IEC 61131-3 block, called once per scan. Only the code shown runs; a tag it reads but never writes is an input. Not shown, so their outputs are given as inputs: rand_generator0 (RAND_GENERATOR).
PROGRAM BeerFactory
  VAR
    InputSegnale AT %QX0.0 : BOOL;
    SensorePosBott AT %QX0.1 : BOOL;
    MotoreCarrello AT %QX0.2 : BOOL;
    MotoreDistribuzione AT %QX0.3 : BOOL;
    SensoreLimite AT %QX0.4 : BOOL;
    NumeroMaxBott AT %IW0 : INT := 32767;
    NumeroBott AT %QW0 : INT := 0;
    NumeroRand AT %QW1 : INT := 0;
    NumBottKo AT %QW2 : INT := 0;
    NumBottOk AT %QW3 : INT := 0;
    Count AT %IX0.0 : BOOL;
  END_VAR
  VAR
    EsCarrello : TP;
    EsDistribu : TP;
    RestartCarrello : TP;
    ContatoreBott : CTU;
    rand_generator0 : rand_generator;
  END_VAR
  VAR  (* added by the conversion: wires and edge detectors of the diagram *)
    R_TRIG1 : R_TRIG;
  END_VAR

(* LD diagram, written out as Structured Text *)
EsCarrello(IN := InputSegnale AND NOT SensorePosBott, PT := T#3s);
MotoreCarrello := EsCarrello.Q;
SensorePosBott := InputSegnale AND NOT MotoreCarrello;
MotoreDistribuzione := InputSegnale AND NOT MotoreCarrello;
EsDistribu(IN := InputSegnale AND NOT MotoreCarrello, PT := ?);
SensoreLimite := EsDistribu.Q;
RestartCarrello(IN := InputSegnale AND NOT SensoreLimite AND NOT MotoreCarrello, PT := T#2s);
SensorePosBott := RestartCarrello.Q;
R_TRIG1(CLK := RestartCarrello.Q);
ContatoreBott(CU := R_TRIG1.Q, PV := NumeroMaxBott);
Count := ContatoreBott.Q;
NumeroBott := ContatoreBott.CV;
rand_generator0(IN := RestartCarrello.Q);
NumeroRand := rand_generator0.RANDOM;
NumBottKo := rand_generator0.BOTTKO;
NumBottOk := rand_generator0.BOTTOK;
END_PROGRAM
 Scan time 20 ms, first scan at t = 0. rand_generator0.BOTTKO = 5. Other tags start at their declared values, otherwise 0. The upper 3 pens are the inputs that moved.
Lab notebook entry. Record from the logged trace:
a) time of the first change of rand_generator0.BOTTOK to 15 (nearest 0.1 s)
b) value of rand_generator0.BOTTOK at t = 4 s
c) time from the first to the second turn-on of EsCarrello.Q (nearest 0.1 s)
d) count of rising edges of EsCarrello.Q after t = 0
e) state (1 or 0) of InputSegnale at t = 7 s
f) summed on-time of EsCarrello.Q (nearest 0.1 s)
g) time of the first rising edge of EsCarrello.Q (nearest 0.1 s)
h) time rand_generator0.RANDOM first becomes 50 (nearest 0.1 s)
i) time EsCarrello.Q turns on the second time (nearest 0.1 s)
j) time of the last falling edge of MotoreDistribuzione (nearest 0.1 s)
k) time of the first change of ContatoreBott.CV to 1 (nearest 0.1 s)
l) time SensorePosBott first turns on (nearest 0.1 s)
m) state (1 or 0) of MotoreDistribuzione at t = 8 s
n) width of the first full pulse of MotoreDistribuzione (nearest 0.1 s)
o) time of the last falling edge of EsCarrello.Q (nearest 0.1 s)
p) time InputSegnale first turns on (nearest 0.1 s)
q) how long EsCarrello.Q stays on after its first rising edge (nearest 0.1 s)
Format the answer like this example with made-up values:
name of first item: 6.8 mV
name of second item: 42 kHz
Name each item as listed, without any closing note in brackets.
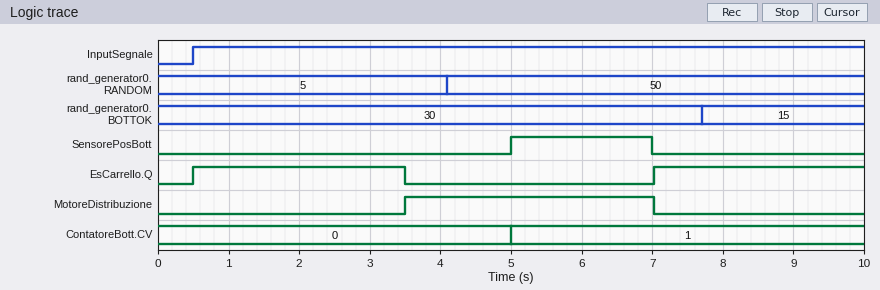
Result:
time of the first change of rand_generator0.BOTTOK to 15: 7.7 s
value of rand_generator0.BOTTOK at t = 4 s: 30
time from the first to the second turn-on of EsCarrello.Q: 6.5 s
count of rising edges of EsCarrello.Q after t = 0: 2
state (1 or 0) of InputSegnale at t = 7 s: 1
summed on-time of EsCarrello.Q: 6.0 s
time of the first rising edge of EsCarrello.Q: 0.5 s
time rand_generator0.RANDOM first becomes 50: 4.1 s
time EsCarrello.Q turns on the second time: 7.0 s
time of the last falling edge of MotoreDistribuzione: 7.0 s
time of the first change of ContatoreBott.CV to 1: 5.0 s
time SensorePosBott first turns on: 5.0 s
state (1 or 0) of MotoreDistribuzione at t = 8 s: 0
width of the first full pulse of MotoreDistribuzione: 3.5 s
time of the last falling edge of EsCarrello.Q: 3.5 s
time InputSegnale first turns on: 0.5 s
how long EsCarrello.Q stays on after its first rising edge: 3.0 s
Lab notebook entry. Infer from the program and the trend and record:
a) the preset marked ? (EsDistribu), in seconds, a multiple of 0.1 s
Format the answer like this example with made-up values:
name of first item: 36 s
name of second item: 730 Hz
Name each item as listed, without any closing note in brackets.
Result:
the preset marked ? (EsDistribu), in seconds, a multiple of 0.1 s: 1.5 s
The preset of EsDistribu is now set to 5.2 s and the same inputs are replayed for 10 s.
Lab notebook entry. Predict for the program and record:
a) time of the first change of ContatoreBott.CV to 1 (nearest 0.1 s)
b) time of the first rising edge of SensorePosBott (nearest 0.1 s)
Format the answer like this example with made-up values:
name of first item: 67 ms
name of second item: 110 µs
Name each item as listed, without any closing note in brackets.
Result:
time of the first change of ContatoreBott.CV to 1: 8.7 s
time of the first rising edge of SensorePosBott: 8.7 s
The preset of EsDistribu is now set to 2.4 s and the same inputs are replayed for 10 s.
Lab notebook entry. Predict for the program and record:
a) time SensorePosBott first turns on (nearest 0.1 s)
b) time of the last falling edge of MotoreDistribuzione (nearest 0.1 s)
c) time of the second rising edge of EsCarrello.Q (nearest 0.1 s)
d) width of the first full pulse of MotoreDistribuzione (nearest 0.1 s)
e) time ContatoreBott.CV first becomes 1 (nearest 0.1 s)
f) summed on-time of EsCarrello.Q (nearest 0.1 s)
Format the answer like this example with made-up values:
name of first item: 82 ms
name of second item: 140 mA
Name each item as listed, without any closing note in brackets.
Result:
time SensorePosBott first turns on: 5.9 s
time of the last falling edge of MotoreDistribuzione: 7.9 s
time of the second rising edge of EsCarrello.Q: 7.9 s
width of the first full pulse of MotoreDistribuzione: 4.4 s
time ContatoreBott.CV first becomes 1: 5.9 s
summed on-time of EsCarrello.Q: 5.1 s
